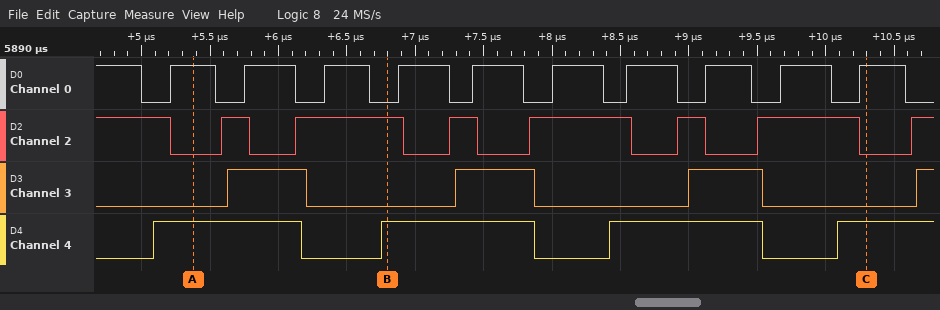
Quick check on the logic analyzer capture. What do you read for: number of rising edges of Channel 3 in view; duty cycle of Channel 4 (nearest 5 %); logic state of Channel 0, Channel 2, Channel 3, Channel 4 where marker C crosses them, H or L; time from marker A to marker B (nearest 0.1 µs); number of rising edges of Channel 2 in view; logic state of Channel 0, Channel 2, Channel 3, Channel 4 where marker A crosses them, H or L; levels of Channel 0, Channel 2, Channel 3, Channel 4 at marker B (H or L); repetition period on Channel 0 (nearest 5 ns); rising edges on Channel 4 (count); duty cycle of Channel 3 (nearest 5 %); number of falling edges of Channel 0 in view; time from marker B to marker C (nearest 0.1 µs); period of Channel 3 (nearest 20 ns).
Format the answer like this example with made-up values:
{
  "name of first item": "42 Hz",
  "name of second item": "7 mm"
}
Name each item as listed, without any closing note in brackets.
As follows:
{
  "number of rising edges of Channel 3 in view": "4",
  "duty cycle of Channel 4": "65 %",
  "logic state of Channel 0, Channel 2, Channel 3, Channel 4 where marker C crosses them, H or L": "Channel 0=H, Channel 2=L, Channel 3=L, Channel 4=H",
  "time from marker A to marker B": "1.4 µs",
  "number of rising edges of Channel 2 in view": "7",
  "logic state of Channel 0, Channel 2, Channel 3, Channel 4 where marker A crosses them, H or L": "Channel 0=H, Channel 2=L, Channel 3=L, Channel 4=H",
  "levels of Channel 0, Channel 2, Channel 3, Channel 4 at marker B": "Channel 0=L, Channel 2=H, Channel 3=L, Channel 4=H",
  "repetition period on Channel 0": "560 ns",
  "rising edges on Channel 4": "4",
  "duty cycle of Channel 3": "35 %",
  "number of falling edges of Channel 0 in view": "11",
  "time from marker B to marker C": "3.5 µs",
  "period of Channel 3": "1680 ns"
}
